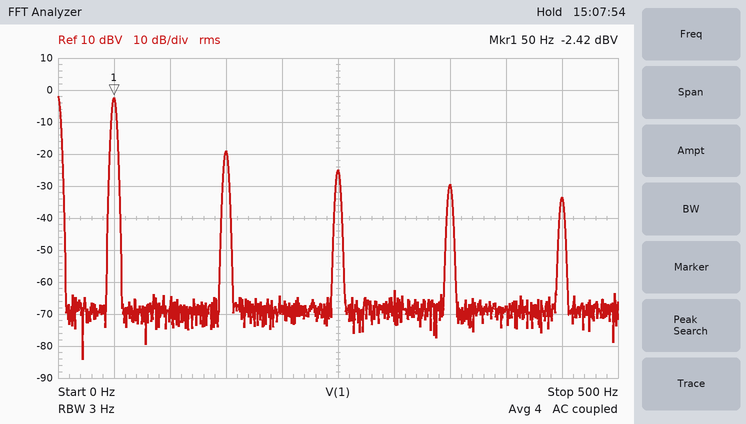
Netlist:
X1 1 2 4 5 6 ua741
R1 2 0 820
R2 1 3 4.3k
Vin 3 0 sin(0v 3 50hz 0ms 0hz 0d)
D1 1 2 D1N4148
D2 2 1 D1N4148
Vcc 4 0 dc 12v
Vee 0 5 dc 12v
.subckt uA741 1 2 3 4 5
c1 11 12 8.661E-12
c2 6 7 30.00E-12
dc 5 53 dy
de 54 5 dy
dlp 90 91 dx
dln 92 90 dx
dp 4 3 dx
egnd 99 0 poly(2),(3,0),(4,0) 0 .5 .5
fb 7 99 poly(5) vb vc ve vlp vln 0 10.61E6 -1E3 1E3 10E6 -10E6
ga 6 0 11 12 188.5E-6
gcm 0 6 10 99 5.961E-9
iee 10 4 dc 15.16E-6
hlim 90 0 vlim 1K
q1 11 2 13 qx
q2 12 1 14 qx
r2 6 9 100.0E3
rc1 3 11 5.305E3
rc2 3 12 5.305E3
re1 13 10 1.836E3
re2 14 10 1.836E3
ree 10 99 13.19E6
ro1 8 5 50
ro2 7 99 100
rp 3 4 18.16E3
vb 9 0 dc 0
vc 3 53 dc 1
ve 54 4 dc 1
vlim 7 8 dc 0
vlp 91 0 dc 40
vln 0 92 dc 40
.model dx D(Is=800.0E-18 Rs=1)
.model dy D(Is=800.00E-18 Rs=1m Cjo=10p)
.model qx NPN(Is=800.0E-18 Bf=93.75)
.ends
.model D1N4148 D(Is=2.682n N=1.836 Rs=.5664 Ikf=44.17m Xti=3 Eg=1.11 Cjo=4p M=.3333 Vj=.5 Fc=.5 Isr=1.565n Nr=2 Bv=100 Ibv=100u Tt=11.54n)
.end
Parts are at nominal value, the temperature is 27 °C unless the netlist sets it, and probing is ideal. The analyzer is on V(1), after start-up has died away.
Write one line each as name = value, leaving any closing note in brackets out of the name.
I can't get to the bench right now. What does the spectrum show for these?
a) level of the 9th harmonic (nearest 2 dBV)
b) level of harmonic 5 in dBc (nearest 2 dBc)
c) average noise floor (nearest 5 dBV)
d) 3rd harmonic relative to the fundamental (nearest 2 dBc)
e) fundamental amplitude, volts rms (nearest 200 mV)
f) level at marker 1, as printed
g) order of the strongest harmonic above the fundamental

level of the 9th harmonic = -34 dBV
level of harmonic 5 in dBc = -22 dBc
average noise floor = -70 dBV
3rd harmonic relative to the fundamental = -16 dBc
fundamental amplitude, volts rms = 800 mV
level at marker 1, as printed = -2.42 dBV
order of the strongest harmonic above the fundamental = 3
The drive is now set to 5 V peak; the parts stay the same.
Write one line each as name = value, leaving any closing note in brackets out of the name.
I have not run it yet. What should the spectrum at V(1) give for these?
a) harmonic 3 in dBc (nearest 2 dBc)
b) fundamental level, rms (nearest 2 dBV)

harmonic 3 in dBc = -18 dBc
fundamental level, rms = 0 dBV
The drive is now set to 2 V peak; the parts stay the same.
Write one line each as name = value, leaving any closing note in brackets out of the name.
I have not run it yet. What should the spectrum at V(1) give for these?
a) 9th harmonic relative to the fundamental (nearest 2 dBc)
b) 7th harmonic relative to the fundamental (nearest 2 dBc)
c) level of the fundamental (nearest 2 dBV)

9th harmonic relative to the fundamental = -34 dBc
7th harmonic relative to the fundamental = -28 dBc
level of the fundamental = -4 dBV
